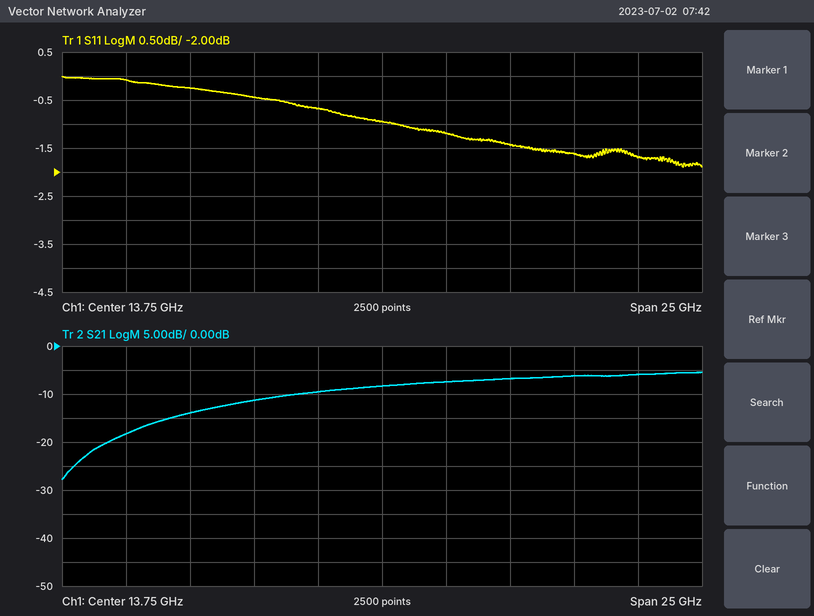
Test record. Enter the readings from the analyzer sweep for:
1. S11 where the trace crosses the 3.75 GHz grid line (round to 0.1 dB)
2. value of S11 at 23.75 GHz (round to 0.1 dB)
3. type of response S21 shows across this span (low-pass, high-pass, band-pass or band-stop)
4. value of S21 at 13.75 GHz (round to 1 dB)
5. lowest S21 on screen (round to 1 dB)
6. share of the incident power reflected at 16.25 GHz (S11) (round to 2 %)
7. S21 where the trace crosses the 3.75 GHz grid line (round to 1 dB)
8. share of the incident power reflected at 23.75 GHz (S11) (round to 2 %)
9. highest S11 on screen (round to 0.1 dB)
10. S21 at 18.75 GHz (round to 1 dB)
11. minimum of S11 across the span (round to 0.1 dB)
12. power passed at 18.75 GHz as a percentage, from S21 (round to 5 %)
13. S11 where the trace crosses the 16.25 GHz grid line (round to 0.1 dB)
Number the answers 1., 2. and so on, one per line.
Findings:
1. -0.1 dB
2. -1.7 dB
3. high-pass
4. -8 dB
5. -28 dB
6. 76 %
7. -18 dB
8. 68 %
9. 0.0 dB
10. -7 dB
11. -1.9 dB
12. 20 %
13. -1.2 dB
